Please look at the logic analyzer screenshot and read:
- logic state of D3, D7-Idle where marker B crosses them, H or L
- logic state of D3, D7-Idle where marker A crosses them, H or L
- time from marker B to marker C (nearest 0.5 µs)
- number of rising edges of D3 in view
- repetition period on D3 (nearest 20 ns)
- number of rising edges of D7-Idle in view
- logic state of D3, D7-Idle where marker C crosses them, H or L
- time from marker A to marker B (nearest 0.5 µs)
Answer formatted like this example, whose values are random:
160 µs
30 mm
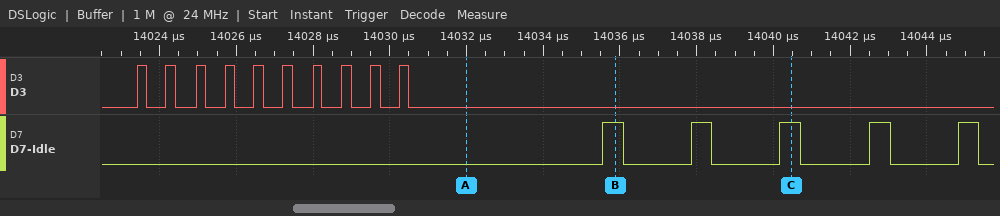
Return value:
D3=L, D7-Idle=H
D3=L, D7-Idle=L
4.5 µs
10
760 ns
5
D3=L, D7-Idle=H
4 µs
